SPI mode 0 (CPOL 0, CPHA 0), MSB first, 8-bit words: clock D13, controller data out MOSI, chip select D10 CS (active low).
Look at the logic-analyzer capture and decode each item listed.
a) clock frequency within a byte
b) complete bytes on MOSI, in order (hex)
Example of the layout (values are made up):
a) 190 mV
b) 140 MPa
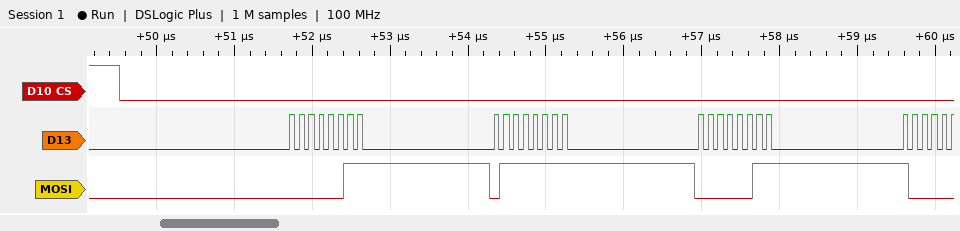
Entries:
a) 8 MHz
b) 03 7F 03
